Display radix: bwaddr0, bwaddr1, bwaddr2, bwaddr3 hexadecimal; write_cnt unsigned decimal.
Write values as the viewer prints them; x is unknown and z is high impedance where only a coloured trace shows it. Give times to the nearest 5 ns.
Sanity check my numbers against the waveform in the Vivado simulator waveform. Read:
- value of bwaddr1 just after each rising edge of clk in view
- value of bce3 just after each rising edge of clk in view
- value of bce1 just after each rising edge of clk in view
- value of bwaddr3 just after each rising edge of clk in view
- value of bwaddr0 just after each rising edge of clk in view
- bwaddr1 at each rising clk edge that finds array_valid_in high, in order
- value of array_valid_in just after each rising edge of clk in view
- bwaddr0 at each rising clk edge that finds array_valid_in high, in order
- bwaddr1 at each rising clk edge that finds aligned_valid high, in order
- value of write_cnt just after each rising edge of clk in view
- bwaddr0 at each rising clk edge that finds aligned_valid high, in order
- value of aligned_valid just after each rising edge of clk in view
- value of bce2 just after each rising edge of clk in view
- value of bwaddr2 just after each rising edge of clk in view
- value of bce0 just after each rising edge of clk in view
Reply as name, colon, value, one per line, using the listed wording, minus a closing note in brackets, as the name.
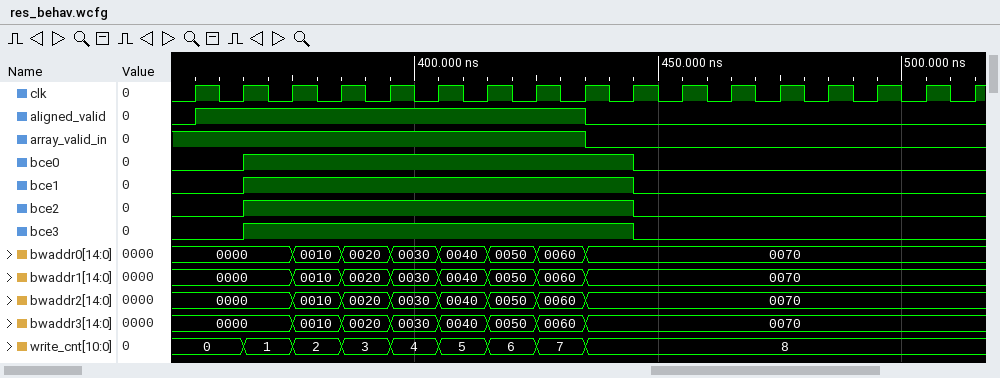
value of bwaddr1 just after each rising edge of clk in view: 0000, 0000, 0010, 0020, 0030, 0040, 0050, 0060, 0070, 0070, 0070, 0070, 0070, 0070, 0070, 0070, 0070
value of bce3 just after each rising edge of clk in view: 0 1 1 1 1 1 1 1 1 0 0 0 0 0 0 0 0
value of bce1 just after each rising edge of clk in view: 0 1 1 1 1 1 1 1 1 0 0 0 0 0 0 0 0
value of bwaddr3 just after each rising edge of clk in view: 0000, 0000, 0010, 0020, 0030, 0040, 0050, 0060, 0070, 0070, 0070, 0070, 0070, 0070, 0070, 0070, 0070
value of bwaddr0 just after each rising edge of clk in view: 0000, 0000, 0010, 0020, 0030, 0040, 0050, 0060, 0070, 0070, 0070, 0070, 0070, 0070, 0070, 0070, 0070
bwaddr1 at each rising clk edge that finds array_valid_in high, in order: 0000, 0000, 0000, 0010, 0020, 0030, 0040, 0050, 0060
value of array_valid_in just after each rising edge of clk in view: 1 1 1 1 1 1 1 1 0 0 0 0 0 0 0 0 0
bwaddr0 at each rising clk edge that finds array_valid_in high, in order: 0000, 0000, 0000, 0010, 0020, 0030, 0040, 0050, 0060
bwaddr1 at each rising clk edge that finds aligned_valid high, in order: 0000, 0000, 0010, 0020, 0030, 0040, 0050, 0060
value of write_cnt just after each rising edge of clk in view: 0, 1, 2, 3, 4, 5, 6, 7, 8, 8, 8, 8, 8, 8, 8, 8, 8
bwaddr0 at each rising clk edge that finds aligned_valid high, in order: 0000, 0000, 0010, 0020, 0030, 0040, 0050, 0060
value of aligned_valid just after each rising edge of clk in view: 1 1 1 1 1 1 1 1 0 0 0 0 0 0 0 0 0
value of bce2 just after each rising edge of clk in view: 0 1 1 1 1 1 1 1 1 0 0 0 0 0 0 0 0
value of bwaddr2 just after each rising edge of clk in view: 0000, 0000, 0010, 0020, 0030, 0040, 0050, 0060, 0070, 0070, 0070, 0070, 0070, 0070, 0070, 0070, 0070
value of bce0 just after each rising edge of clk in view: 0 1 1 1 1 1 1 1 1 0 0 0 0 0 0 0 0
